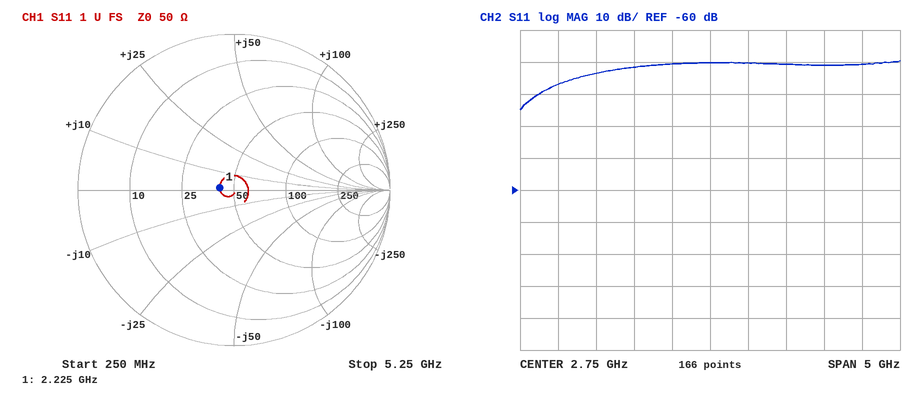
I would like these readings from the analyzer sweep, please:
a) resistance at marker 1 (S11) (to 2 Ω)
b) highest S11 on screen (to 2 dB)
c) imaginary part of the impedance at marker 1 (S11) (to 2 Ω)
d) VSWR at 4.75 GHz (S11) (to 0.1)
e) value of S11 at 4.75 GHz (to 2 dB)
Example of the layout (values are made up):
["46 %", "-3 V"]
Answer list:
["42 Ω", "-20 dB", "+2 Ω", "1.2", "-20 dB"]
